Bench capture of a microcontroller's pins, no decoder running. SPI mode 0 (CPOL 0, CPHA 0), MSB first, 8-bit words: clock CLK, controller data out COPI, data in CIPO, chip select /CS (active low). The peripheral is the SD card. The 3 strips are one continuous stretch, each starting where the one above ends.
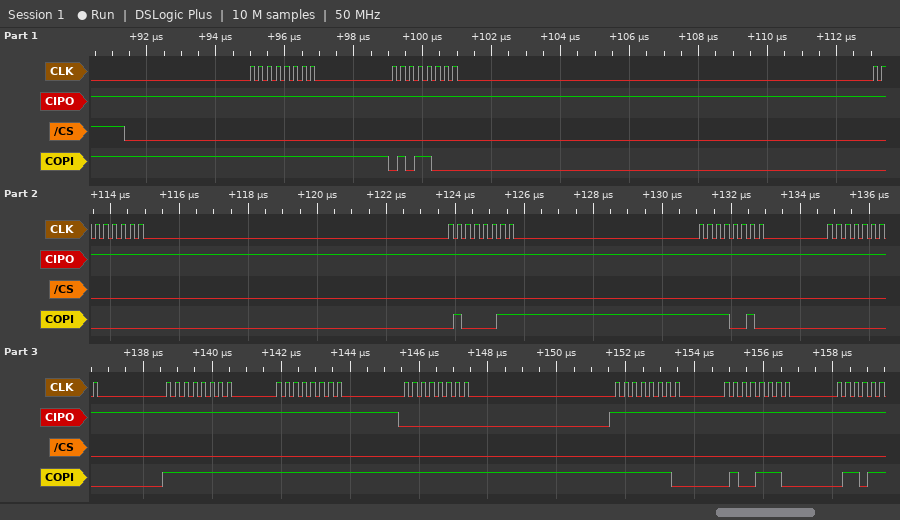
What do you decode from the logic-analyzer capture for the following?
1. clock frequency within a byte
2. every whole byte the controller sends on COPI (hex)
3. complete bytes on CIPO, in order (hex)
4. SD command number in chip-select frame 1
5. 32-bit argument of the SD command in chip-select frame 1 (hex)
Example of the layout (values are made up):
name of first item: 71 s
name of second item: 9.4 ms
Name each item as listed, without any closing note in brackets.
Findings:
clock frequency within a byte: 4 MHz
every whole byte the controller sends on COPI: 0xFF 0x58 0x00 0x43 0xF2 0x00 0xFF 0xFF 0xFF 0xFE 0x4E
complete bytes on CIPO, in order: 0xFF 0xFF 0xFF 0xFF 0xFF 0xFF 0xFF 0xFF 0x00 0xFF 0xFF
SD command number in chip-select frame 1: CMD24
32-bit argument of the SD command in chip-select frame 1: 0x0043F200
